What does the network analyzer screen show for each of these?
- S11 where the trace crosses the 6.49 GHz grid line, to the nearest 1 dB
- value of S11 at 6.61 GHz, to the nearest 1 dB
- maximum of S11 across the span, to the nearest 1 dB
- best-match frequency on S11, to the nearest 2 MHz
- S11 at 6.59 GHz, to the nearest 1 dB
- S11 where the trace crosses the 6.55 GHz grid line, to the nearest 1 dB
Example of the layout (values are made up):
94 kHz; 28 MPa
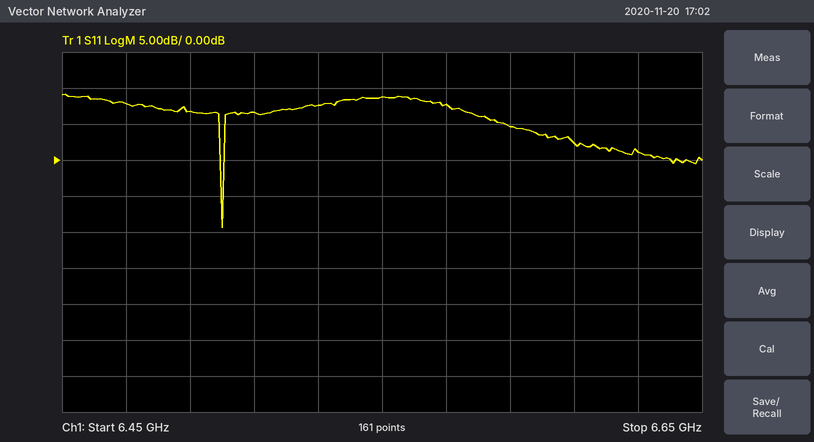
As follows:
7 dB; 2 dB; 9 dB; 6.500 GHz; 5 dB; 9 dB
